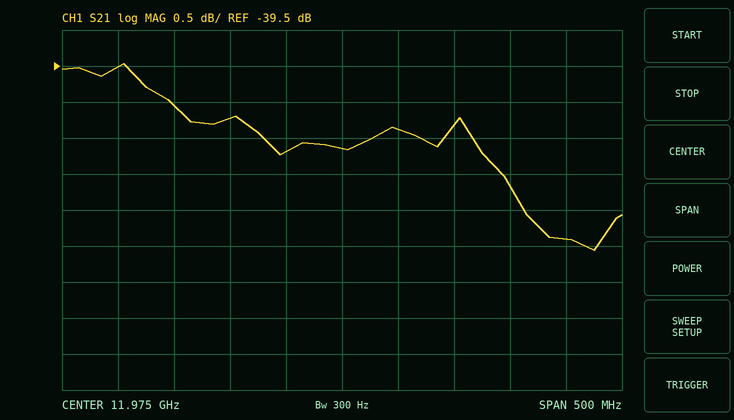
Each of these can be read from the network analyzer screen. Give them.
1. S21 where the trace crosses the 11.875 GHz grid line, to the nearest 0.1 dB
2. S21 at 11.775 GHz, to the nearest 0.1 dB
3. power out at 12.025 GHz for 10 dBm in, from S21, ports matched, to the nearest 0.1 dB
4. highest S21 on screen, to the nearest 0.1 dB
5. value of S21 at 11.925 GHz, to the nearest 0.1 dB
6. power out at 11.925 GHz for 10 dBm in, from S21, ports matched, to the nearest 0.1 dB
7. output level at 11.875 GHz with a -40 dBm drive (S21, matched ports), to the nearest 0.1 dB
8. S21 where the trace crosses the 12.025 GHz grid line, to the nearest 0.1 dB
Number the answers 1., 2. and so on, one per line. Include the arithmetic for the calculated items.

1. -40.2 dB
2. -39.5 dB
3. 10 dBm + (-40.4 dB) = -30.4 dBm
4. -39.5 dB
5. -40.7 dB
6. 10 dBm + (-40.7 dB) = -30.7 dBm
7. -40 dBm + (-40.2 dB) = -80.2 dBm
8. -40.4 dB
